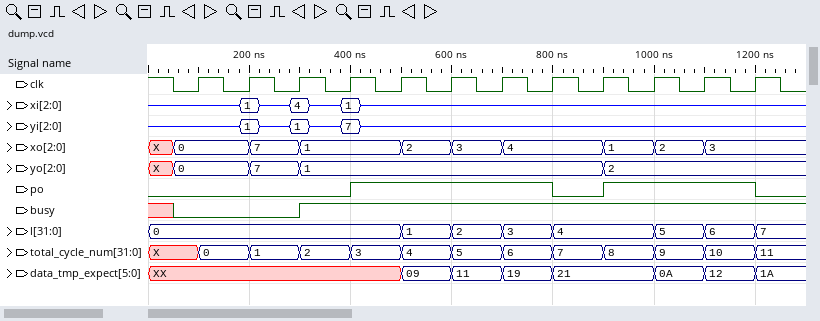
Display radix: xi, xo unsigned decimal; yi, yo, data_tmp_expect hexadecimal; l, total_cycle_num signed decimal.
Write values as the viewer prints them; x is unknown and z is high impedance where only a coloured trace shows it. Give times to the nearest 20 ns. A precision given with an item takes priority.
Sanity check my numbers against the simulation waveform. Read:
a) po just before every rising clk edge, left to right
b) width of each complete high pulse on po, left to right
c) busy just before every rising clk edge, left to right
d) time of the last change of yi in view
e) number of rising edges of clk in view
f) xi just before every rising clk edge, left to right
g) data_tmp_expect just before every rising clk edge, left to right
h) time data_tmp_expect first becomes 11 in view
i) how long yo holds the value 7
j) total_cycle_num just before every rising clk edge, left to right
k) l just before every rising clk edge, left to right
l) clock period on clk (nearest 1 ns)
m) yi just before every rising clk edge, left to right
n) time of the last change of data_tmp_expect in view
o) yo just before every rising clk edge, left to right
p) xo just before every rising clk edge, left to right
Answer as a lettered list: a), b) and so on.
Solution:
a) 0 0 0 0 1 1 1 1 0 1 1 1
b) 400 ns, 300 ns
c) 0 0 0 1 1 1 1 1 1 1 1 1
d) 420 ns
e) 12
f) z, 1, 4, 1, z, z, z, z, z, z, z, z
g) XX, XX, XX, XX, XX, 09, 11, 19, 21, 21, 0A, 12
h) 600 ns
i) 100 ns
j) X, 0, 1, 2, 3, 4, 5, 6, 7, 8, 9, 10
k) 0, 0, 0, 0, 0, 1, 2, 3, 4, 4, 5, 6
l) 100 ns
m) z, 1, 1, 7, z, z, z, z, z, z, z, z
n) 1200 ns
o) 0, 0, 7, 1, 1, 1, 1, 1, 1, 2, 2, 2
p) 0, 0, 7, 1, 1, 2, 3, 4, 4, 1, 2, 3
